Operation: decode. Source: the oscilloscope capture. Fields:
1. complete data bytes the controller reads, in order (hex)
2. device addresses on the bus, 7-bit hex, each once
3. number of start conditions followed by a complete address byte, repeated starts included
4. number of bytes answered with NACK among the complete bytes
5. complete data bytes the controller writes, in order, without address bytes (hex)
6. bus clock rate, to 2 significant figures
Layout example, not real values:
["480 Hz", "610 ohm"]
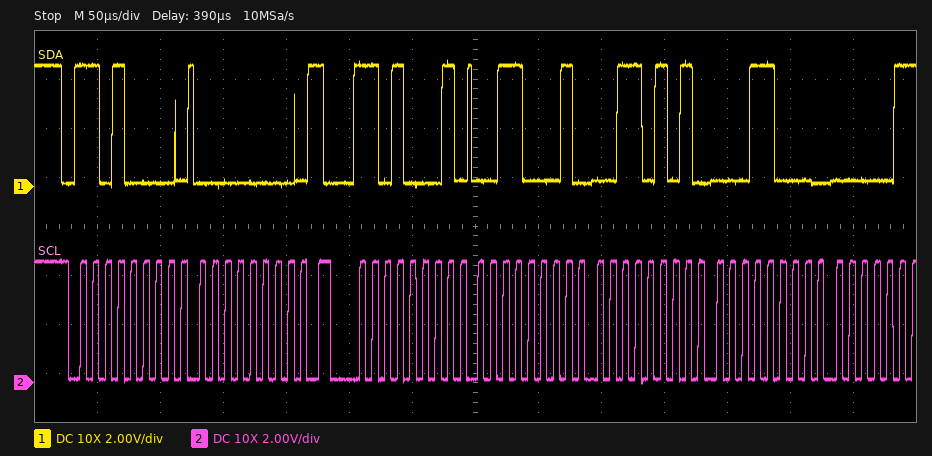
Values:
["31 35 18", "0x68", "2", "0", "00", "100 kHz"]
